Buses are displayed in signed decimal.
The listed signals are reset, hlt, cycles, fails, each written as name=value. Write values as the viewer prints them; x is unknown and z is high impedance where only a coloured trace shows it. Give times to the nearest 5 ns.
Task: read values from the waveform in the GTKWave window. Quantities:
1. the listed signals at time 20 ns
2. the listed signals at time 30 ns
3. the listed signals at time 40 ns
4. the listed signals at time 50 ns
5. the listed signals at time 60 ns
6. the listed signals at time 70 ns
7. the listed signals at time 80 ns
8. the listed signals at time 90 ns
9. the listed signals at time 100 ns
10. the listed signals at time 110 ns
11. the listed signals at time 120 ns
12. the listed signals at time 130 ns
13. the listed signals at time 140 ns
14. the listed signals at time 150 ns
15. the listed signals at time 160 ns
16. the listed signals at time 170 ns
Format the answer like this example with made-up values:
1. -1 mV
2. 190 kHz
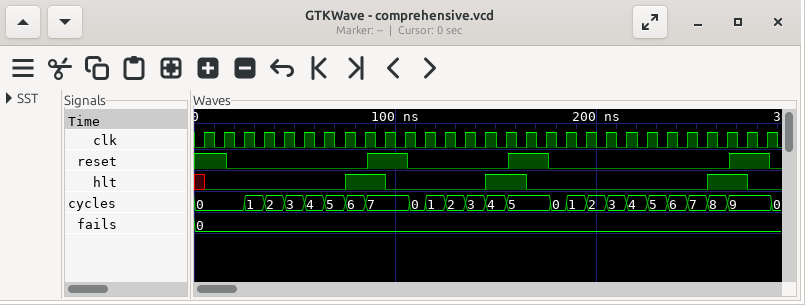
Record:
1. reset=0, hlt=0, cycles=0, fails=0
2. reset=0, hlt=0, cycles=1, fails=0
3. reset=0, hlt=0, cycles=2, fails=0
4. reset=0, hlt=0, cycles=3, fails=0
5. reset=0, hlt=0, cycles=4, fails=0
6. reset=0, hlt=0, cycles=5, fails=0
7. reset=0, hlt=1, cycles=6, fails=0
8. reset=1, hlt=1, cycles=7, fails=0
9. reset=1, hlt=0, cycles=7, fails=0
10. reset=0, hlt=0, cycles=0, fails=0
11. reset=0, hlt=0, cycles=1, fails=0
12. reset=0, hlt=0, cycles=2, fails=0
13. reset=0, hlt=0, cycles=3, fails=0
14. reset=0, hlt=1, cycles=4, fails=0
15. reset=1, hlt=1, cycles=5, fails=0
16. reset=1, hlt=0, cycles=5, fails=0
